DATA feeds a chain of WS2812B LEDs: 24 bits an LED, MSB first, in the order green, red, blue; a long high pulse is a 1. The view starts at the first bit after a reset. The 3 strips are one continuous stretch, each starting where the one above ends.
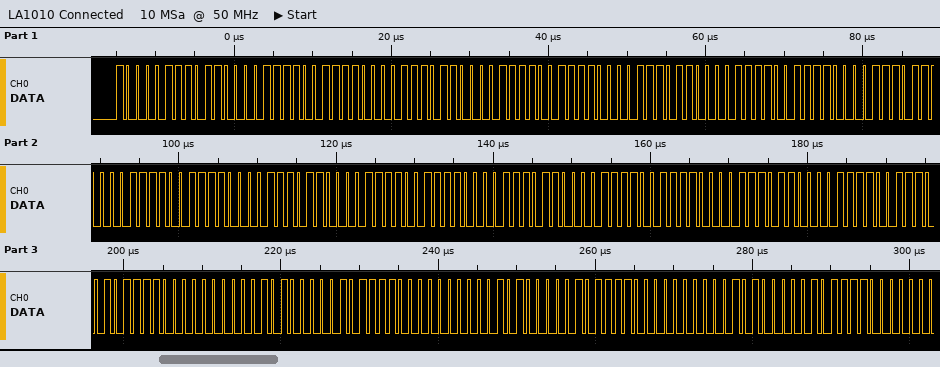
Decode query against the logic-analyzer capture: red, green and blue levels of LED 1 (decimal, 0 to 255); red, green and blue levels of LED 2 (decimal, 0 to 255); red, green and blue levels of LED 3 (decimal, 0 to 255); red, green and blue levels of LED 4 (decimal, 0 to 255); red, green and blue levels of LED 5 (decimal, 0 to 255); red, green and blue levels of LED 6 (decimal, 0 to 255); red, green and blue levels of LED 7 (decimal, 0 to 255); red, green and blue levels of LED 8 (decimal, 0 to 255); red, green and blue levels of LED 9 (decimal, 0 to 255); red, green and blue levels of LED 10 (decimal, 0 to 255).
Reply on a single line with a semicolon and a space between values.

97, 135, 231; 97, 135, 231; 97, 135, 231; 97, 135, 231; 97, 135, 231; 97, 135, 231; 97, 135, 231; 0, 47, 40; 0, 47, 40; 0, 47, 40
